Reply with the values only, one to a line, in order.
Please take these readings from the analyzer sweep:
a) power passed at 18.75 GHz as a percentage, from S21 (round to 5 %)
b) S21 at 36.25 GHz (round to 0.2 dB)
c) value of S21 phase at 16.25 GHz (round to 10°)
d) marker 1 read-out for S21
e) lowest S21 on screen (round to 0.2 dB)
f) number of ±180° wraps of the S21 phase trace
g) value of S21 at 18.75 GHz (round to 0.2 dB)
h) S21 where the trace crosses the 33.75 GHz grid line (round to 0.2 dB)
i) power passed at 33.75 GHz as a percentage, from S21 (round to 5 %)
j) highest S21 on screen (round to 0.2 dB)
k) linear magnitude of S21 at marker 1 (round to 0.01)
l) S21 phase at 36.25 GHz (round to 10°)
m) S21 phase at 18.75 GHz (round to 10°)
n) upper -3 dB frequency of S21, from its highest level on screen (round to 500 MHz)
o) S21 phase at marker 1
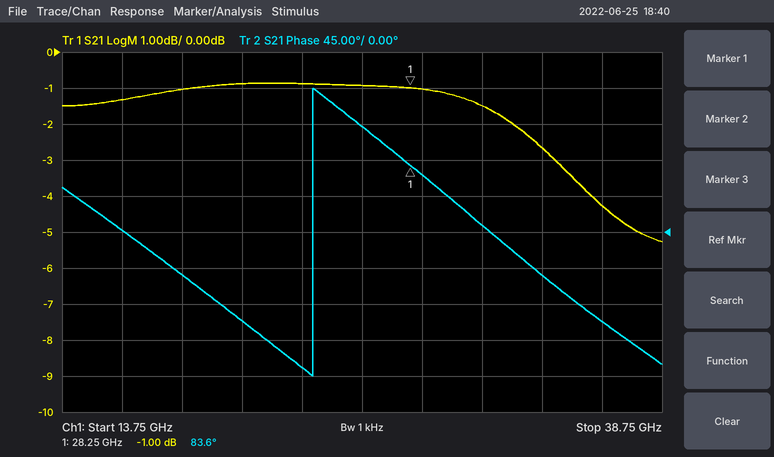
80 %
-4.2 dB
0°
-1.00 dB
-5.2 dB
1
-1.0 dB
-2.6 dB
55 %
-0.8 dB
0.89
-110°
-50°
35.5 GHz
83.6°
